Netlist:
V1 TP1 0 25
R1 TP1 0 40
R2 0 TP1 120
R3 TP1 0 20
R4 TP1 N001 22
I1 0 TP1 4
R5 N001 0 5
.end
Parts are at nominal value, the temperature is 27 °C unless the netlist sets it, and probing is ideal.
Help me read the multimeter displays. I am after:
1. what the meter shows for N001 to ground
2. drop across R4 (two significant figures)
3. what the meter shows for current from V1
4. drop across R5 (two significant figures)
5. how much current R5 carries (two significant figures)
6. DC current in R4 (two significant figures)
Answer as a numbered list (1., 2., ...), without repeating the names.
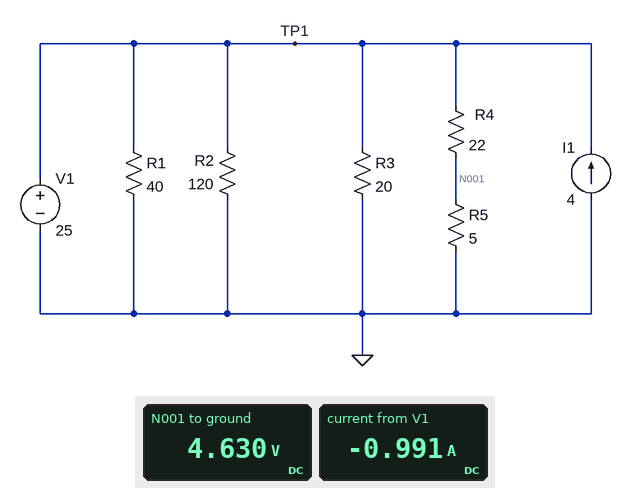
1. 4.630 V
2. 20 V
3. -0.991 A
4. 4.6 V
5. 930 mA
6. 930 mA
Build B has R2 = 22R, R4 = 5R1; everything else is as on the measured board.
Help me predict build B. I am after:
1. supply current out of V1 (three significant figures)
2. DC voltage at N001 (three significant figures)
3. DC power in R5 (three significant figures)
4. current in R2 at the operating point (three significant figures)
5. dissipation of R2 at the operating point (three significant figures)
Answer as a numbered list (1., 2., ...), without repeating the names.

1. 1.49 A
2. 12.4 V
3. 30.6 W
4. 1.14 A
5. 28.4 W
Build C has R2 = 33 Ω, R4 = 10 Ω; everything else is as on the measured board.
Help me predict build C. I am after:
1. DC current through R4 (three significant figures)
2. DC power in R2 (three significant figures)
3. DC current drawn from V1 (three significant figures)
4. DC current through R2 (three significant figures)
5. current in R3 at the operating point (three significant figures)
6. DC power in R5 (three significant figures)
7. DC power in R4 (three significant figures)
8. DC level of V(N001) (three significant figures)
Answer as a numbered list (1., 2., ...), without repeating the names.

1. 1.67 A
2. 18.9 W
3. 299 mA
4. 758 mA
5. 1.25 A
6. 13.9 W
7. 27.8 W
8. 8.33 V
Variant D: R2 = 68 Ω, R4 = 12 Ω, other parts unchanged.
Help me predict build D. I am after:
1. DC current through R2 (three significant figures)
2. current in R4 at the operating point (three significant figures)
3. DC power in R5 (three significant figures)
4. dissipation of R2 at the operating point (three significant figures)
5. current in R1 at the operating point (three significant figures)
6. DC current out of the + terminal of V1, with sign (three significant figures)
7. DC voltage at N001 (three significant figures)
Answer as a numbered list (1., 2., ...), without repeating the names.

1. 368 mA
2. 1.47 A
3. 10.8 W
4. 9.19 W
5. 625 mA
6. -287 mA
7. 7.35 V
